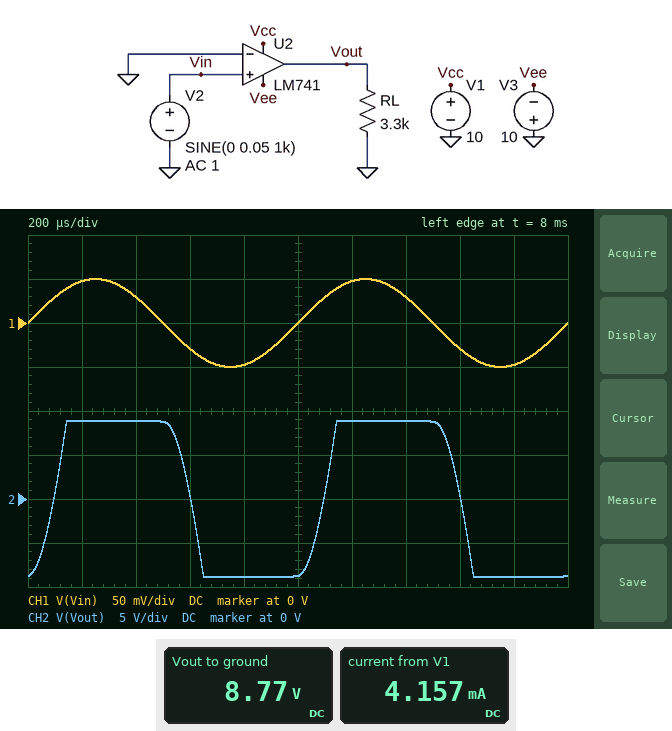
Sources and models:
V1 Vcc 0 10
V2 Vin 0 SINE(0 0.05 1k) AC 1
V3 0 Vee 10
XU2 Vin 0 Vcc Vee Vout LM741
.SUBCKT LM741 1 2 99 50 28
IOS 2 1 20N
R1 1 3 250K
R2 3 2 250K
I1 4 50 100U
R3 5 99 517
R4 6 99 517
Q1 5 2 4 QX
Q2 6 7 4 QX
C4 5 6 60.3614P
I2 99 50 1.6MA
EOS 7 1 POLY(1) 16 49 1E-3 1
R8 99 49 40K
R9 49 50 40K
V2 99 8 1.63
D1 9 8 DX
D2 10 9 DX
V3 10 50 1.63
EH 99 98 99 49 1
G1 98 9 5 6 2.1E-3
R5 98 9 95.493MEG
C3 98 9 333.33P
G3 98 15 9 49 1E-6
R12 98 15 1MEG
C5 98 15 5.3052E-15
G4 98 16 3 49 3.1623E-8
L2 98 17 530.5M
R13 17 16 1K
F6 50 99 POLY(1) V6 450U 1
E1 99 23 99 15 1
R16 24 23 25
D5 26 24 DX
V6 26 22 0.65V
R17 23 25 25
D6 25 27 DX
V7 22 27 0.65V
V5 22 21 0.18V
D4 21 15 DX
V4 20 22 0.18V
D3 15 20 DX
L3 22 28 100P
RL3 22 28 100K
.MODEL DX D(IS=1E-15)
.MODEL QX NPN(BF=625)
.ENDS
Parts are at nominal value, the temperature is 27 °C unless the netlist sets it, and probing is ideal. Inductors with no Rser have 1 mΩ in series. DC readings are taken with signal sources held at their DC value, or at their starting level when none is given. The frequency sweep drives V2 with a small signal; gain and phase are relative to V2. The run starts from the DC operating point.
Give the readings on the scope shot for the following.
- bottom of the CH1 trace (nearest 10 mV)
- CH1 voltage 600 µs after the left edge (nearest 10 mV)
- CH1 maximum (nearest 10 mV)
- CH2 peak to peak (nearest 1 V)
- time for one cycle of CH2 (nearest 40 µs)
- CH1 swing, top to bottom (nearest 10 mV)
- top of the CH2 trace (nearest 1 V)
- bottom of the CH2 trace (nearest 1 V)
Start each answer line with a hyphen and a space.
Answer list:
- -50 mV
- -30 mV
- 50 mV
- 18 V
- 1.00 ms
- 100 mV
- 9 V
- -9 V
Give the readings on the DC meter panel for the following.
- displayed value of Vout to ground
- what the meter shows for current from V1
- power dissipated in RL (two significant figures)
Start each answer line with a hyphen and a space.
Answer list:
- 8.77 V
- 4.157 mA
- 23 mW
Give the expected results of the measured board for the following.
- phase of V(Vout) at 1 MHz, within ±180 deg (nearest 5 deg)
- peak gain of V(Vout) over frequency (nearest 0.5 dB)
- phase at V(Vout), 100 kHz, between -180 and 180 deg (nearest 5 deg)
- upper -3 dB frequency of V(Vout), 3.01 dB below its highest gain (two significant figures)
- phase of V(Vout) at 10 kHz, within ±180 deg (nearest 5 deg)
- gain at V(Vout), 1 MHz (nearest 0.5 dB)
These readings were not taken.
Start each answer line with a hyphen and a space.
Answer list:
- -110 deg
- 28.5 dB
- -70 deg
- 37 kHz
- -15 deg
- -0.5 dB
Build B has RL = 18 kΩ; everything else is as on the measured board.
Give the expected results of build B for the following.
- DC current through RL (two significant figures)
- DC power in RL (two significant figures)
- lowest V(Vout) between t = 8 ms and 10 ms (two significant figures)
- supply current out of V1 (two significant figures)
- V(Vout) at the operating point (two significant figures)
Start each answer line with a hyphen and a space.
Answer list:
- 490 µA
- 4.4 mW
- -9.0 V
- 2.0 mA
- 8.9 V
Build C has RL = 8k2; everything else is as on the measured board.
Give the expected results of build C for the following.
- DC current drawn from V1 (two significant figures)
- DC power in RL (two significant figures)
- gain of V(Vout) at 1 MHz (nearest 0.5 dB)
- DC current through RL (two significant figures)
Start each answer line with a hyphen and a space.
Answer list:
- 2.6 mA
- 9.5 mW
- -0.5 dB
- 1.1 mA
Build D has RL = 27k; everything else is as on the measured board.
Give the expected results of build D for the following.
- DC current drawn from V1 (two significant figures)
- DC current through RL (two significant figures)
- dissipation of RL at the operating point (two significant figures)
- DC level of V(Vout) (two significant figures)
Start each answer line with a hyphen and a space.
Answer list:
- 1.8 mA
- 330 µA
- 2.9 mW
- 8.9 V
